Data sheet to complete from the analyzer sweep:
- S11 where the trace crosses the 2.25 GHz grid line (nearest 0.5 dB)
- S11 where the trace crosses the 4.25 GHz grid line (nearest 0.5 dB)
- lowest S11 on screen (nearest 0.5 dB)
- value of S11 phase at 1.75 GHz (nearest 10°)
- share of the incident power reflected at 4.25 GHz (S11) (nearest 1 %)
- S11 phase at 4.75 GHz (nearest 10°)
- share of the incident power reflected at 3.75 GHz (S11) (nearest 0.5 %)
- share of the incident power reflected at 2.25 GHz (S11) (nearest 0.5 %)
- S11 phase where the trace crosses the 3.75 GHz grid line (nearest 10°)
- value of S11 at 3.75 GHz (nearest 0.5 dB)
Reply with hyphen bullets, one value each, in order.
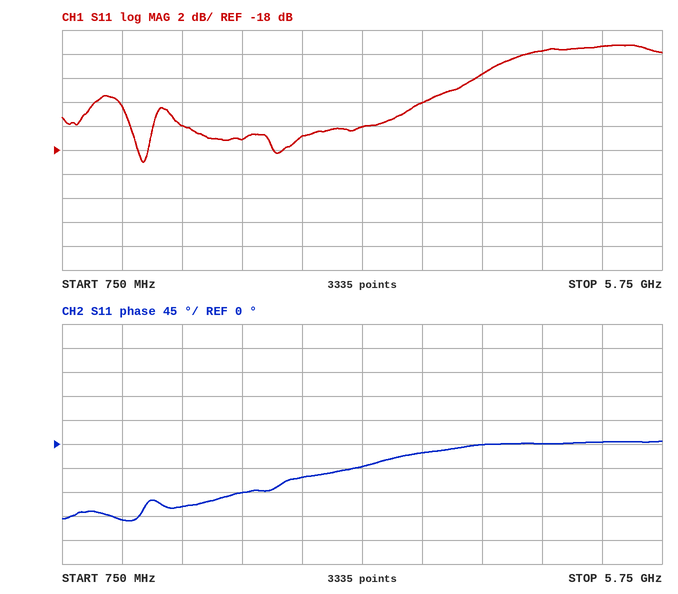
- -17.0 dB
- -11.5 dB
- -19.0 dB
- -120°
- 7 %
- 0°
- 4.0 %
- 2.0 %
- -20°
- -14.0 dB
